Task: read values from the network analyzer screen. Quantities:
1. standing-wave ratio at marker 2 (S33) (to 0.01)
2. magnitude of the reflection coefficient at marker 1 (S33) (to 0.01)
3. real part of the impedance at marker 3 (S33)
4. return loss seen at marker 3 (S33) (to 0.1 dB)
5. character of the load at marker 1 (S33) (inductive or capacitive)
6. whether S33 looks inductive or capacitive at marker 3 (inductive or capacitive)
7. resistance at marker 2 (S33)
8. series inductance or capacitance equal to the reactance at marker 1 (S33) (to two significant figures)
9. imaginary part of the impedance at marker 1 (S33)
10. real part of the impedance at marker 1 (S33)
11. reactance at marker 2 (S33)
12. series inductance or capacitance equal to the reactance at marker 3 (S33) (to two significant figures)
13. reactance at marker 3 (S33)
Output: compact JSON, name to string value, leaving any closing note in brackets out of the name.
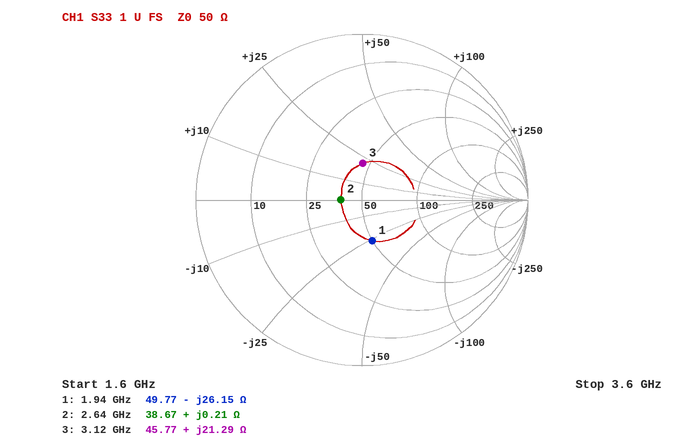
{"standing-wave ratio at marker 2 (S33)": "1.29", "magnitude of the reflection coefficient at marker 1 (S33)": "0.25", "real part of the impedance at marker 3": "45.77 Ω", "return loss seen at marker 3 (S33)": "13.1 dB", "character of the load at marker 1 (S33)": "capacitive", "whether S33 looks inductive or capacitive at marker 3": "inductive", "resistance at marker 2": "38.67 Ω", "series inductance or capacitance equal to the reactance at marker 1 (S33)": "3.1 pF", "imaginary part of the impedance at marker 1": "-26.15 Ω", "real part of the impedance at marker 1": "49.77 Ω", "reactance at marker 2": "+0.21 Ω", "series inductance or capacitance equal to the reactance at marker 3 (S33)": "1.1 nH", "reactance at marker 3": "+21.29 Ω"}
